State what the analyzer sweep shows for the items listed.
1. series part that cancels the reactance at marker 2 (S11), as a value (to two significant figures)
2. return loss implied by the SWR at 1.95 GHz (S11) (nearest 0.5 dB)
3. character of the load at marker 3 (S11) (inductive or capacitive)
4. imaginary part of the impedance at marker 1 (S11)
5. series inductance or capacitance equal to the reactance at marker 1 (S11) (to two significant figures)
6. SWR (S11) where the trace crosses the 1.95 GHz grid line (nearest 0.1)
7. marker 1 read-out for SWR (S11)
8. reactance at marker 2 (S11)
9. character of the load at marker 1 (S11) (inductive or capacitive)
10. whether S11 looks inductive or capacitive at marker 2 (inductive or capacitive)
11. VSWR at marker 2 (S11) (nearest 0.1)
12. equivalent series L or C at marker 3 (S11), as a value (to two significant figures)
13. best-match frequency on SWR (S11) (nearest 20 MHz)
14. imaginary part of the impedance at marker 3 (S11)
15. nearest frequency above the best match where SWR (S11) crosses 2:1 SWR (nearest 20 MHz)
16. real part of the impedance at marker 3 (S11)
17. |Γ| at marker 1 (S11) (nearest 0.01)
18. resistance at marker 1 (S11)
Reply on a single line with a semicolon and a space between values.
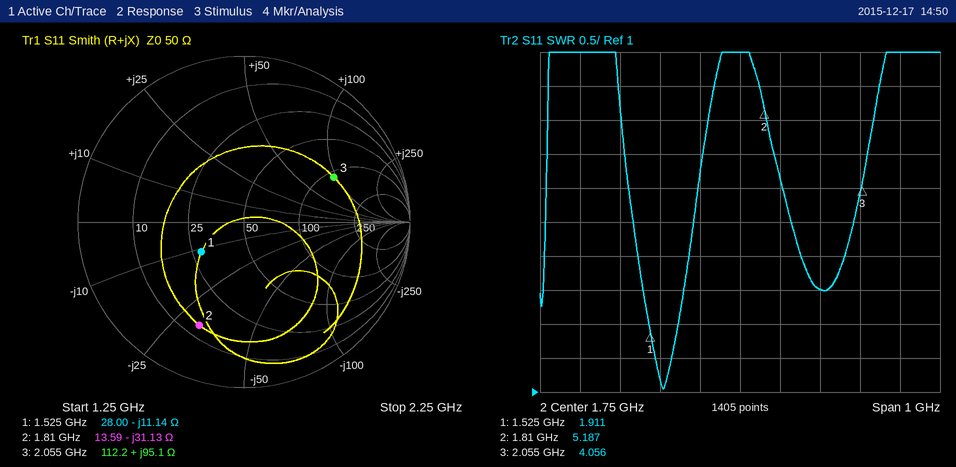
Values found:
2.7 nH; 7.5 dB; inductive; -11.14 Ω; 9.4 pF; 2.5; 1.911; -31.13 Ω; capacitive; capacitive; 5.2; 7.4 nH; 1.56 GHz; +95.1 Ω; 1.60 GHz; 112.2 Ω; 0.31; 28.00 Ω
